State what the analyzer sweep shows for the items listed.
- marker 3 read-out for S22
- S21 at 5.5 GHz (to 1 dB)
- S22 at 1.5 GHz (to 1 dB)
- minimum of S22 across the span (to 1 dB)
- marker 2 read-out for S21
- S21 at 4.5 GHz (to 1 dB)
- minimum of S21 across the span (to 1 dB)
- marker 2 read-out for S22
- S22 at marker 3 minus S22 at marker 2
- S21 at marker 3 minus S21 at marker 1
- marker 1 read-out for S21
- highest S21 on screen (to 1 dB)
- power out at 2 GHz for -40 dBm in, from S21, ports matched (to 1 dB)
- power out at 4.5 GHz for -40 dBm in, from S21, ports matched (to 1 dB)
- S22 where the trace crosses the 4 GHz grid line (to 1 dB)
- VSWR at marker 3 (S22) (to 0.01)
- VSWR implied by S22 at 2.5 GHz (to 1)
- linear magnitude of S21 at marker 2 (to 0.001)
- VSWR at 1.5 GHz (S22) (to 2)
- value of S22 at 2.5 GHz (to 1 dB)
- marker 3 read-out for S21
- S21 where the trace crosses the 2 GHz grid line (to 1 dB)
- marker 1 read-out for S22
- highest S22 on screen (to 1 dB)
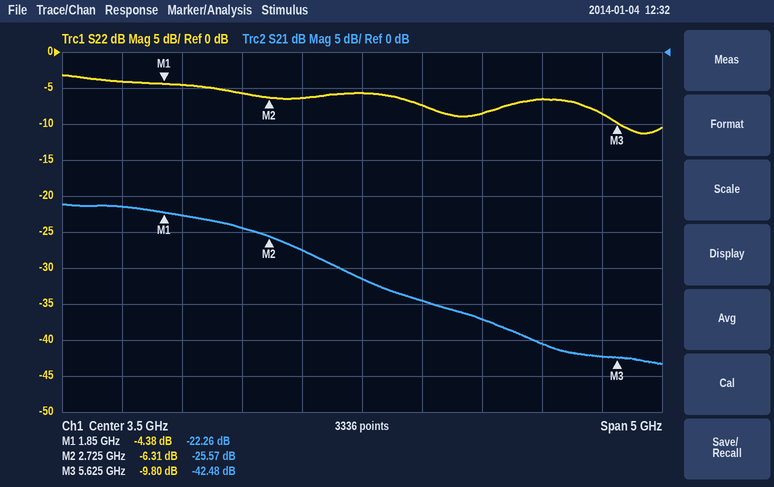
-9.80 dB
-42 dB
-4 dB
-11 dB
-25.57 dB
-37 dB
-43 dB
-6.31 dB
-3.49 dB
-20.22 dB
-22.26 dB
-21 dB
-63 dBm
-77 dBm
-7 dB
1.96
3
0.053
4
-6 dB
-42.48 dB
-23 dB
-4.38 dB
-3 dB
